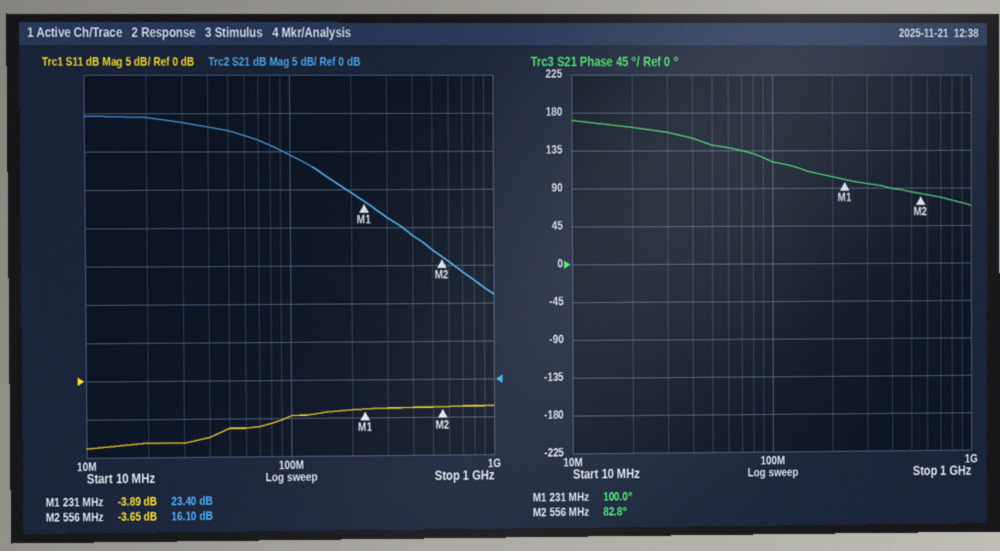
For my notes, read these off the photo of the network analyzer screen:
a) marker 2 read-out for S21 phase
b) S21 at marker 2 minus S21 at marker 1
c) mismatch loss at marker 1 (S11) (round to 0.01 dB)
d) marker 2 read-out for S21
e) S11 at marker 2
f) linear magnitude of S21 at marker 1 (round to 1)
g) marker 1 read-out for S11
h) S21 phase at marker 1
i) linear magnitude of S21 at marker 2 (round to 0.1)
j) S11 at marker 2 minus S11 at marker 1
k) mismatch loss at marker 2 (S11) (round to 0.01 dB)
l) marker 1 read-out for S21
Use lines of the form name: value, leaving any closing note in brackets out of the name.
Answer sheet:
marker 2 read-out for S21 phase: 82.8°
S21 at marker 2 minus S21 at marker 1: -7.30 dB
mismatch loss at marker 1 (S11): 2.28 dB
marker 2 read-out for S21: 16.10 dB
S11 at marker 2: -3.65 dB
linear magnitude of S21 at marker 1: 15
marker 1 read-out for S11: -3.89 dB
S21 phase at marker 1: 100.0°
linear magnitude of S21 at marker 2: 6.4
S11 at marker 2 minus S11 at marker 1: 0.24 dB
mismatch loss at marker 2 (S11): 2.45 dB
marker 1 read-out for S21: 23.40 dB
